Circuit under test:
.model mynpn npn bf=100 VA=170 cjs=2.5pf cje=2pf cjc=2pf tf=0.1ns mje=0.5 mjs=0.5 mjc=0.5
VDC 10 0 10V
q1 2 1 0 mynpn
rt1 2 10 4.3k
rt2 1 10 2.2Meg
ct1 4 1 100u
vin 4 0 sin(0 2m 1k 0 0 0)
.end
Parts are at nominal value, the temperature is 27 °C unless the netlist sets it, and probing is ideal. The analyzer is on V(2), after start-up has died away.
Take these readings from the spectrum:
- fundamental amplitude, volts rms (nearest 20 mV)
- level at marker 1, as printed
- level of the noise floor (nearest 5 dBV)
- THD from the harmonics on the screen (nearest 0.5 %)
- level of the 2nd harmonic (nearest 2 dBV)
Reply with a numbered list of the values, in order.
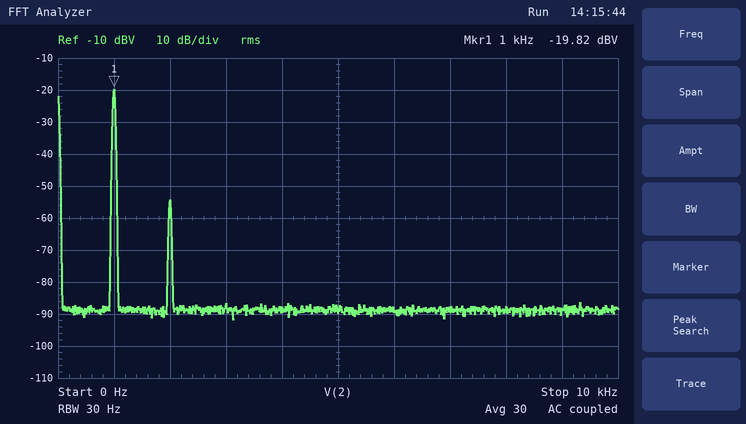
1. 100 mV
2. -19.82 dBV
3. -90 dBV
4. 2.0 %
5. -54 dBV
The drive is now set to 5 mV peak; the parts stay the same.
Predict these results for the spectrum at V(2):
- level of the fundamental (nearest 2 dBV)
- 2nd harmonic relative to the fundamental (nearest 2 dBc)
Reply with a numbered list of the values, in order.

1. -12 dBV
2. -26 dBc
